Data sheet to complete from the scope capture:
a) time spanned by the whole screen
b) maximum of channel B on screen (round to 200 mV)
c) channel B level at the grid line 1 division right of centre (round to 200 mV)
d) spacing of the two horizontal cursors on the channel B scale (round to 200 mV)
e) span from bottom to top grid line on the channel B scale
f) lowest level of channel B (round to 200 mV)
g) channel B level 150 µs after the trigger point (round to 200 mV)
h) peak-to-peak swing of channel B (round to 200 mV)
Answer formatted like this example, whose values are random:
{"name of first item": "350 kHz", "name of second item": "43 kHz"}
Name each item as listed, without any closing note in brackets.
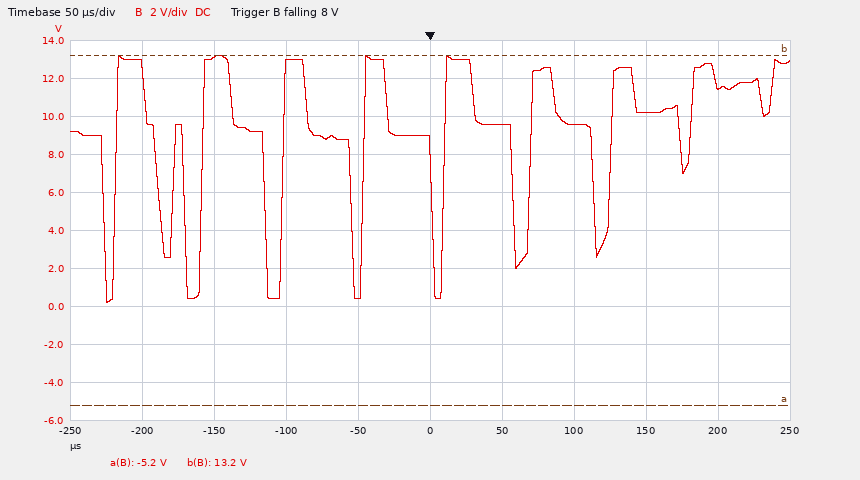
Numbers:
{"time spanned by the whole screen": "500 µs", "maximum of channel B on screen": "13.2 V", "channel B level at the grid line 1 division right of centre": "9.6 V", "spacing of the two horizontal cursors on the channel B scale": "18.4 V", "span from bottom to top grid line on the channel B scale": "20 V", "lowest level of channel B": "200 mV", "channel B level 150 µs after the trigger point": "10.2 V", "peak-to-peak swing of channel B": "13.0 V"}
